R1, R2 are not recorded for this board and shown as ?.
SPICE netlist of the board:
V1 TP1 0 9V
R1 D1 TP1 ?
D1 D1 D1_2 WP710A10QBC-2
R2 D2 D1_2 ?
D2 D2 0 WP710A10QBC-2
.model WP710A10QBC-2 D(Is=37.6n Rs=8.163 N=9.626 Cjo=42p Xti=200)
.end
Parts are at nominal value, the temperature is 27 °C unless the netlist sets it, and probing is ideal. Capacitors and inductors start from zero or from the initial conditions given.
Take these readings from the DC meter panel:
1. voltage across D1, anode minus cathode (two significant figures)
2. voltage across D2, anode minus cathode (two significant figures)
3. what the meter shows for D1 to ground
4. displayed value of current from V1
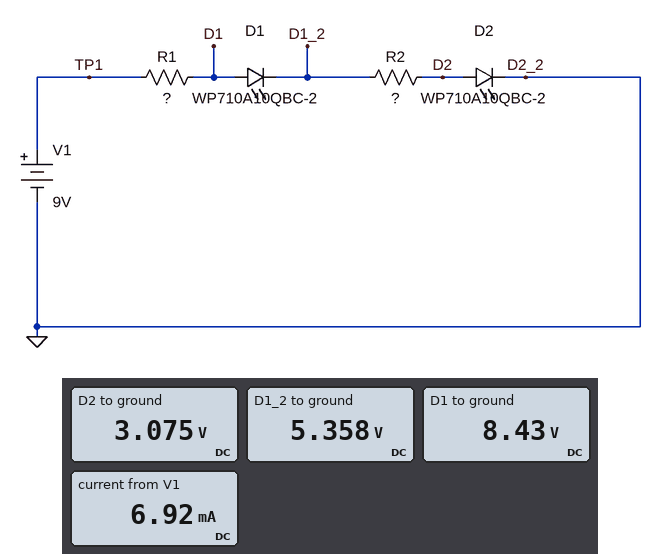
3.1 V
3.1 V
8.43 V
6.92 mA
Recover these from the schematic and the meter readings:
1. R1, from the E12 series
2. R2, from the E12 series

82 Ω
330 Ω
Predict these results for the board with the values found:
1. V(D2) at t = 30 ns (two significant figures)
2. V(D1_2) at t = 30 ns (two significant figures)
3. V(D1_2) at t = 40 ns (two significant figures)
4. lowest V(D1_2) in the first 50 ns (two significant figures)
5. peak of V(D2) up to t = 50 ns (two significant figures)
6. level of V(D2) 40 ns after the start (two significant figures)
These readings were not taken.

2.9 V
5.5 V
5.4 V
5.4 V
3.1 V
3.0 V
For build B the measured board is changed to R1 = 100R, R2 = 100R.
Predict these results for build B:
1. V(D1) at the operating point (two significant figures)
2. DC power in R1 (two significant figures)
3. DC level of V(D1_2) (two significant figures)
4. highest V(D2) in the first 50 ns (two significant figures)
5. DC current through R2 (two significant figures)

7.8 V
15 mW
4.5 V
3.3 V
12 mA
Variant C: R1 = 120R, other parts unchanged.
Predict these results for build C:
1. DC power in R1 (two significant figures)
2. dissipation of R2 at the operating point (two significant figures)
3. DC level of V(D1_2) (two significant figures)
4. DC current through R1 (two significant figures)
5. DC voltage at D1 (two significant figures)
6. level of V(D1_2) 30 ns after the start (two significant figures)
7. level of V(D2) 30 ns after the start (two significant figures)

5.0 mW
14 mW
5.2 V
6.4 mA
8.2 V
5.3 V
2.8 V
